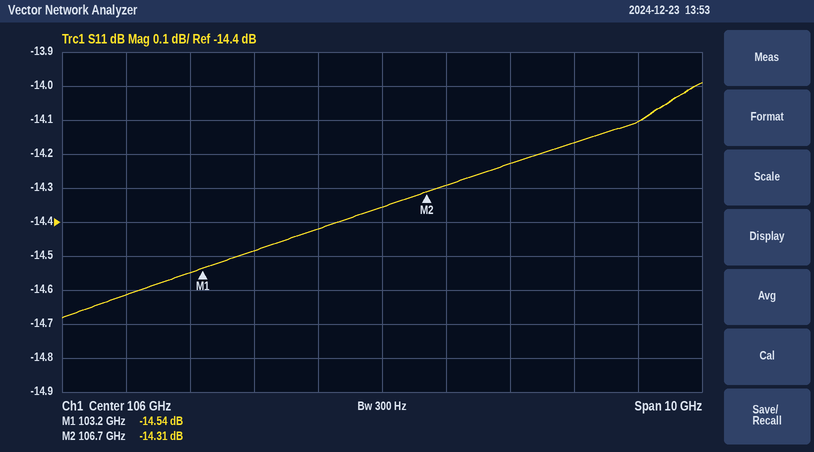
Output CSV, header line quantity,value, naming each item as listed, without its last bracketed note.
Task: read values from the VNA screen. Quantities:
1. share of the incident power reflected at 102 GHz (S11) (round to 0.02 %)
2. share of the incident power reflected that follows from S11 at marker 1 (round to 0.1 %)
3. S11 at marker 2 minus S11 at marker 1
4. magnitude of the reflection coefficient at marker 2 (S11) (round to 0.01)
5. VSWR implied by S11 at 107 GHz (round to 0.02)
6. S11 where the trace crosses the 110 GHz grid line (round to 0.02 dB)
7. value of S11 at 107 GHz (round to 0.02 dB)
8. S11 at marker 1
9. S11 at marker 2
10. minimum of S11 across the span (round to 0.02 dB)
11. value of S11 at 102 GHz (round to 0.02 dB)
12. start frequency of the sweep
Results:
quantity,value
share of the incident power reflected at 102 GHz (S11),3.46 %
share of the incident power reflected that follows from S11 at marker 1,3.5 %
S11 at marker 2 minus S11 at marker 1,0.23 dB
magnitude of the reflection coefficient at marker 2 (S11),0.19
VSWR implied by S11 at 107 GHz,1.48
S11 where the trace crosses the 110 GHz grid line,-14.10 dB
value of S11 at 107 GHz,-14.30 dB
S11 at marker 1,-14.54 dB
S11 at marker 2,-14.31 dB
minimum of S11 across the span,-14.68 dB
value of S11 at 102 GHz,-14.62 dB
start frequency of the sweep,101 GHz
